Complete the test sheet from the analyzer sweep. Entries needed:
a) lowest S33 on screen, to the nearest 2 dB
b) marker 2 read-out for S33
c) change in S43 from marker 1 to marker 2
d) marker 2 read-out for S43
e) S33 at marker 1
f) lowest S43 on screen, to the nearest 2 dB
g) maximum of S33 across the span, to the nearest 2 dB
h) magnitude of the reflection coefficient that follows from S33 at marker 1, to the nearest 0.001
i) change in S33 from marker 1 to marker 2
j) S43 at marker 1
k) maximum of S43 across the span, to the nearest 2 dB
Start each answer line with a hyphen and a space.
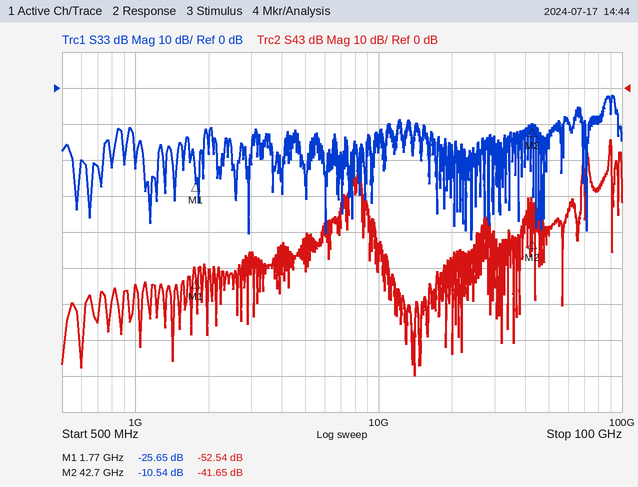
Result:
- -42 dB
- -10.54 dB
- 10.89 dB
- -41.65 dB
- -25.65 dB
- -80 dB
- -2 dB
- 0.052
- 15.11 dB
- -52.54 dB
- -14 dB
